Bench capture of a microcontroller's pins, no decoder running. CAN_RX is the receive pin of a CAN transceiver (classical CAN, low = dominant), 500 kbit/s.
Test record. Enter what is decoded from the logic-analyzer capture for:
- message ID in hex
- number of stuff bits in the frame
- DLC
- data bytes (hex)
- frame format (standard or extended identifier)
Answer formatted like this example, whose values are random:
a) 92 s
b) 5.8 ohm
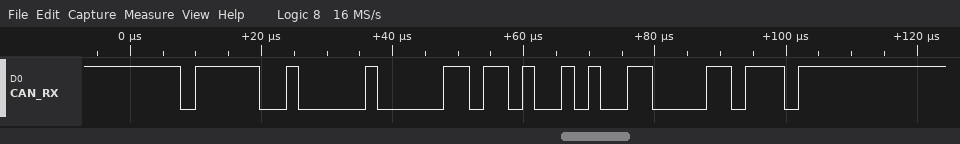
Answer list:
a) 0x7D0
b) 3
c) 1
d) 69
e) standard
